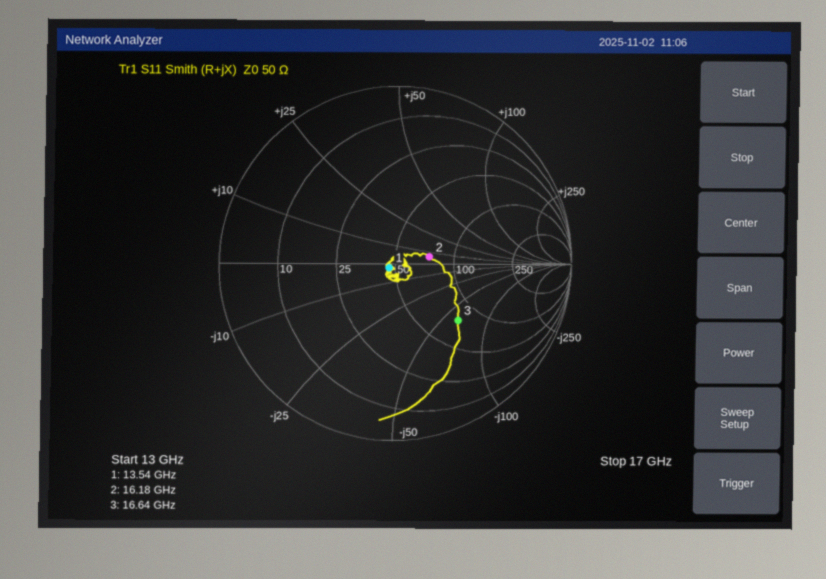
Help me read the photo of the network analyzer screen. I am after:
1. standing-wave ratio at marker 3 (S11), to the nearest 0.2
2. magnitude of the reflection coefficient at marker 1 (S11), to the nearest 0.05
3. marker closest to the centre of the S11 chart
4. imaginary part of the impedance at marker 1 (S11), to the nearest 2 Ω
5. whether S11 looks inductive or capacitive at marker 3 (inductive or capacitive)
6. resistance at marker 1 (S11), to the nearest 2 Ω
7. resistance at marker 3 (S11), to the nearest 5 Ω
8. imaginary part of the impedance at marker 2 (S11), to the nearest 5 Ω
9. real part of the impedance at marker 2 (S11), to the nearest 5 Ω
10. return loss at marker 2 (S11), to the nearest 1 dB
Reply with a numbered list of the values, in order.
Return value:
1. 2.8
2. 0.05
3. marker 1
4. -2 Ω
5. capacitive
6. 46 Ω
7. 75 Ω
8. +5 Ω
9. 75 Ω
10. 14 dB
